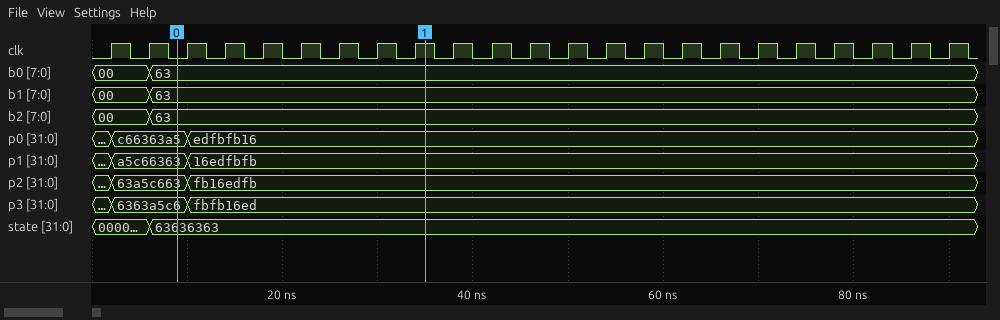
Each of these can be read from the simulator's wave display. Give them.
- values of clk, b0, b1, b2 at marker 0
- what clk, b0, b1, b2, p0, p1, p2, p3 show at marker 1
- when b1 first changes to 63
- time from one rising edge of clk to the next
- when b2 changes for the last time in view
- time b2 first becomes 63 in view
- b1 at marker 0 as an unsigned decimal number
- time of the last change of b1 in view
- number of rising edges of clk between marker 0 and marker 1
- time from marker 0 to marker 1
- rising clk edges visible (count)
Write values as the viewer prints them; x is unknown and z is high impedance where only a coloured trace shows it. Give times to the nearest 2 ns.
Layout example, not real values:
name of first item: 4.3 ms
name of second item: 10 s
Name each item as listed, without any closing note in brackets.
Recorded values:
values of clk, b0, b1, b2 at marker 0: clk=0, b0=63, b1=63, b2=63
what clk, b0, b1, b2, p0, p1, p2, p3 show at marker 1: clk=1, b0=63, b1=63, b2=63, p0=edfbfb16, p1=16edfbfb, p2=fb16edfb, p3=fbfb16ed
when b1 first changes to 63: 6 ns
time from one rising edge of clk to the next: 4 ns
when b2 changes for the last time in view: 6 ns
time b2 first becomes 63 in view: 6 ns
b1 at marker 0 as an unsigned decimal number: 99
time of the last change of b1 in view: 6 ns
number of rising edges of clk between marker 0 and marker 1: 7
time from marker 0 to marker 1: 26 ns
rising clk edges visible: 23
